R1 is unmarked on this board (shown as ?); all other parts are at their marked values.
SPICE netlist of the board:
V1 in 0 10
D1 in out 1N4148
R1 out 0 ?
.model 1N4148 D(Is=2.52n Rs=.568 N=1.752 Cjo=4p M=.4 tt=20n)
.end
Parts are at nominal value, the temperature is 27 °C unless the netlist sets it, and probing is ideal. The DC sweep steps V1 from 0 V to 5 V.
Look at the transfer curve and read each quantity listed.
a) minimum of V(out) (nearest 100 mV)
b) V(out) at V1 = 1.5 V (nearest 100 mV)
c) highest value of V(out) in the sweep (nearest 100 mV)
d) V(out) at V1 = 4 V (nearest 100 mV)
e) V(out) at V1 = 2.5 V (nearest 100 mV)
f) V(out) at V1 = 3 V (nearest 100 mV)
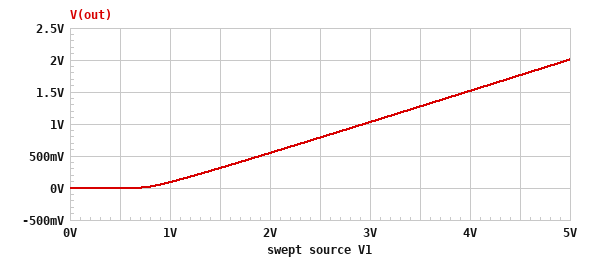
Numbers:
0 V
300 mV
2.0 V
1.5 V
800 mV
1.0 V
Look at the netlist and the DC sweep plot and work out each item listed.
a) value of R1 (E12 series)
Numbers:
0.56 Ω
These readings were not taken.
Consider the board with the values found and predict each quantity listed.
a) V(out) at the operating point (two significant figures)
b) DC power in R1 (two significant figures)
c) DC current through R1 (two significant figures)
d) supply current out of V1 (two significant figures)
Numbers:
4.5 V
36 W
8.0 A
8.0 A
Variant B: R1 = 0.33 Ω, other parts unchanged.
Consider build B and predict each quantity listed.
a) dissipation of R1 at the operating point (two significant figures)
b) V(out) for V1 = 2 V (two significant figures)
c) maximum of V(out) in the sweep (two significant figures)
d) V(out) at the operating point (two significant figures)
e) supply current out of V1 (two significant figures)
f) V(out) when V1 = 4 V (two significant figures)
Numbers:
33 W
400 mV
1.5 V
3.3 V
10 A
1.1 V
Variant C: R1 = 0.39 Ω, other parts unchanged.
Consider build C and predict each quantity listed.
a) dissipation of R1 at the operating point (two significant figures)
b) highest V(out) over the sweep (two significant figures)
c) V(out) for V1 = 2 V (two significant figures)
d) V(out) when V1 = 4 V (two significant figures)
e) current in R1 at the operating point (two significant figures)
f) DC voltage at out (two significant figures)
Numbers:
34 W
1.6 V
450 mV
1.2 V
9.4 A
3.7 V
